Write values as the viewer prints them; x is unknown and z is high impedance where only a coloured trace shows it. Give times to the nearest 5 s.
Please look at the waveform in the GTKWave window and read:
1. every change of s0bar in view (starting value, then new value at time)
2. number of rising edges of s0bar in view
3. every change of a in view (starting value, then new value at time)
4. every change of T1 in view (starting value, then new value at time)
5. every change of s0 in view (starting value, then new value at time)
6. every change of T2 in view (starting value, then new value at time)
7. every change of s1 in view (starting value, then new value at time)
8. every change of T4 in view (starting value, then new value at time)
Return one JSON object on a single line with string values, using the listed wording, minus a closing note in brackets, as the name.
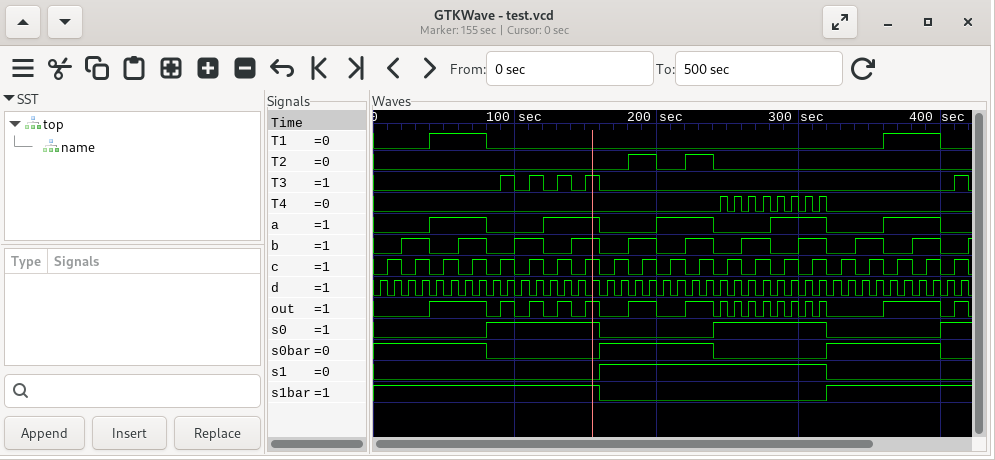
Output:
{"every change of s0bar in view": "1, 0 at 80 s, 1 at 160 s, 0 at 240 s, 1 at 320 s, 0 at 400 s", "number of rising edges of s0bar in view": "2", "every change of a in view": "0, 1 at 40 s, 0 at 80 s, 1 at 120 s, 0 at 160 s, 1 at 200 s, 0 at 240 s, 1 at 280 s, 0 at 320 s, 1 at 360 s, 0 at 400 s", "every change of T1 in view": "0, 1 at 40 s, 0 at 80 s, 1 at 360 s, 0 at 400 s", "every change of s0 in view": "0, 1 at 80 s, 0 at 160 s, 1 at 240 s, 0 at 320 s, 1 at 400 s", "every change of T2 in view": "0, 1 at 180 s, 0 at 200 s, 1 at 220 s, 0 at 240 s", "every change of s1 in view": "0, 1 at 160 s, 0 at 320 s", "every change of T4 in view": "0, 1 at 245 s, 0 at 250 s, 1 at 255 s, 0 at 260 s, 1 at 265 s, 0 at 270 s, 1 at 275 s, 0 at 280 s, 1 at 285 s, 0 at 290 s, 1 at 295 s, 0 at 300 s, 1 at 305 s, 0 at 310 s, 1 at 315 s, 0 at 320 s"}
